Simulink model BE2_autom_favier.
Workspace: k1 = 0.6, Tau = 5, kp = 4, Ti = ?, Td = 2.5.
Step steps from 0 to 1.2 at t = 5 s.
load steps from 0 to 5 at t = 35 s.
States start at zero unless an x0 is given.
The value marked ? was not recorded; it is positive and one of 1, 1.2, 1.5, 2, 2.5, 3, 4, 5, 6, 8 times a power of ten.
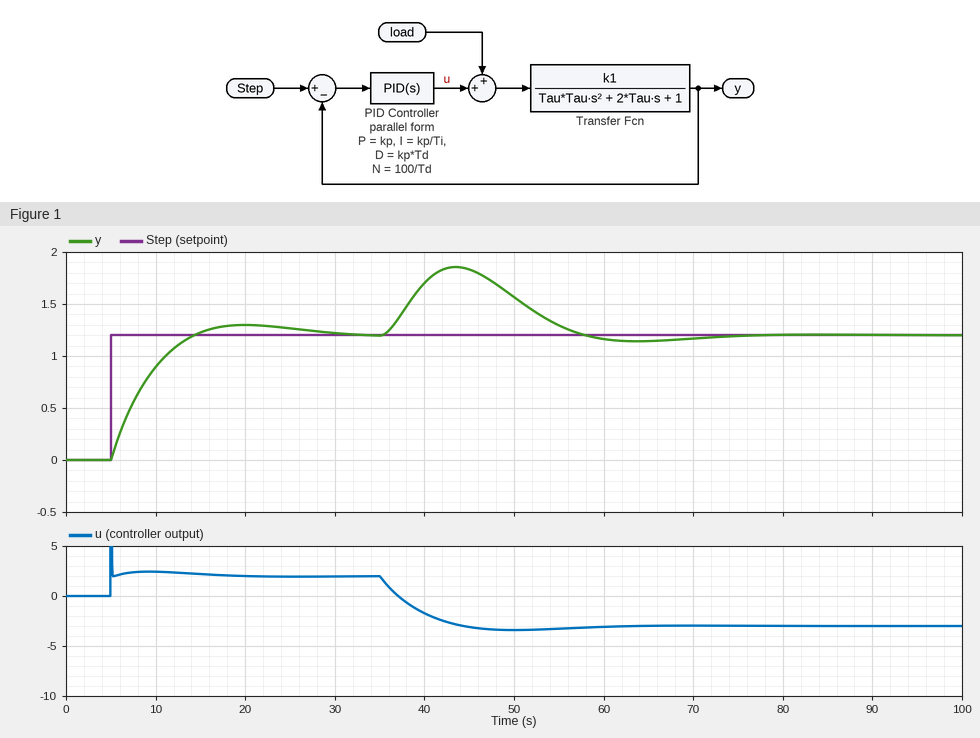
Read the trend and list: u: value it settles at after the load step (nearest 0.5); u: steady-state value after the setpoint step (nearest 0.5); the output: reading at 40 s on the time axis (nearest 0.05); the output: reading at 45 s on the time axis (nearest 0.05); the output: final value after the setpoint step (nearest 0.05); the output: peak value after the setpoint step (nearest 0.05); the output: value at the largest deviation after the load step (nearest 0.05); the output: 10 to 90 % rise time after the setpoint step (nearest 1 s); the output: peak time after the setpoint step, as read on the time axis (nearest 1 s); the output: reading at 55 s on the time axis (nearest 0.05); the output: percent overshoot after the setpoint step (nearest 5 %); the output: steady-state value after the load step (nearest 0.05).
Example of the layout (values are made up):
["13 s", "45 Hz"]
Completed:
["-3.0", "2.0", "1.70", "1.85", "1.20", "1.30", "1.85", "7 s", "20 s", "1.30", "10 %", "1.20"]
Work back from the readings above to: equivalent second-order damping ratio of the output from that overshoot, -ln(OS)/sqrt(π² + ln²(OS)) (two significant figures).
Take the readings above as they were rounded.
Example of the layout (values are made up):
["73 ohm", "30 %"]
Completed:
["0.59"]
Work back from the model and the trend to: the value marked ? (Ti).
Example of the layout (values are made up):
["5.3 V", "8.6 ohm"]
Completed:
["6"]
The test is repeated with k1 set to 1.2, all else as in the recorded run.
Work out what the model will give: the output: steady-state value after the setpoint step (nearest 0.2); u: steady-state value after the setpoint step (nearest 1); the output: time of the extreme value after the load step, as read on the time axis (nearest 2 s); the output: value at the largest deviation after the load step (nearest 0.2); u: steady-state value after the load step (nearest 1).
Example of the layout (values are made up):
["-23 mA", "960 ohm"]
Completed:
["1.2", "1", "42 s", "2.0", "-4"]
